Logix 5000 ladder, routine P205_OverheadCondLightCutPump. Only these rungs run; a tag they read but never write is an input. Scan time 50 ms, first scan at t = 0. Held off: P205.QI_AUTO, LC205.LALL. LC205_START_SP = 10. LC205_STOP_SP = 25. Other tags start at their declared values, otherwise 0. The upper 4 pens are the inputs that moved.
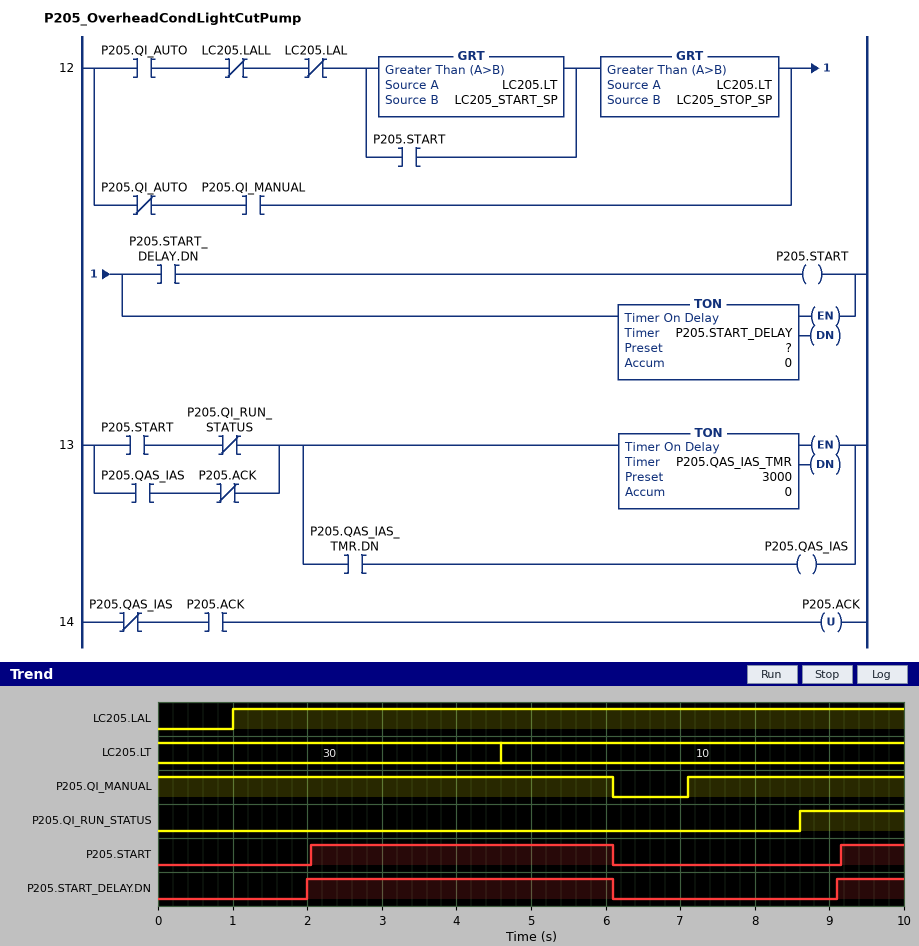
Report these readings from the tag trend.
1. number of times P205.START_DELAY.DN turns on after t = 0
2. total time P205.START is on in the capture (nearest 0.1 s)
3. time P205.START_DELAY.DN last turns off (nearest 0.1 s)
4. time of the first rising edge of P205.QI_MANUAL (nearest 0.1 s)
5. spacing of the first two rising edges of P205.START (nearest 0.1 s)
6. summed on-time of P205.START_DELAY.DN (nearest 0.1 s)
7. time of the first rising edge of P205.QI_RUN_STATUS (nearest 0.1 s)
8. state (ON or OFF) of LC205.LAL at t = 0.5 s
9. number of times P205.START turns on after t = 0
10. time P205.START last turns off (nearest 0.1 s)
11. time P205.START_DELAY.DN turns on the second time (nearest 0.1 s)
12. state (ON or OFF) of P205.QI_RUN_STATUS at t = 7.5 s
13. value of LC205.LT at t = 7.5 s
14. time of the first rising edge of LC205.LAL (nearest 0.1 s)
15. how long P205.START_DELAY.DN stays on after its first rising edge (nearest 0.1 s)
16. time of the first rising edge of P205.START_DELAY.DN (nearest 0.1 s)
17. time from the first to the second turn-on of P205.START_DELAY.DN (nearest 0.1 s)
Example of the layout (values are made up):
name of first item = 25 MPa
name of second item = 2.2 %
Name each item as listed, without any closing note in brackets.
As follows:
number of times P205.START_DELAY.DN turns on after t = 0 = 2
total time P205.START is on in the capture = 4.9 s
time P205.START_DELAY.DN last turns off = 6.1 s
time of the first rising edge of P205.QI_MANUAL = 7.1 s
spacing of the first two rising edges of P205.START = 7.1 s
summed on-time of P205.START_DELAY.DN = 5.0 s
time of the first rising edge of P205.QI_RUN_STATUS = 8.6 s
state (ON or OFF) of LC205.LAL at t = 0.5 s = OFF
number of times P205.START turns on after t = 0 = 2
time P205.START last turns off = 6.1 s
time P205.START_DELAY.DN turns on the second time = 9.1 s
state (ON or OFF) of P205.QI_RUN_STATUS at t = 7.5 s = OFF
value of LC205.LT at t = 7.5 s = 10
time of the first rising edge of LC205.LAL = 1.0 s
how long P205.START_DELAY.DN stays on after its first rising edge = 4.1 s
time of the first rising edge of P205.START_DELAY.DN = 2.0 s
time from the first to the second turn-on of P205.START_DELAY.DN = 7.1 s
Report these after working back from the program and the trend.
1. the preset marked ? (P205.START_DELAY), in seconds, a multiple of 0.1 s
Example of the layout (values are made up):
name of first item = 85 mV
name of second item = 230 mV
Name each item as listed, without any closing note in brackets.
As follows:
the preset marked ? (P205.START_DELAY), in seconds, a multiple of 0.1 s = 2.0 s
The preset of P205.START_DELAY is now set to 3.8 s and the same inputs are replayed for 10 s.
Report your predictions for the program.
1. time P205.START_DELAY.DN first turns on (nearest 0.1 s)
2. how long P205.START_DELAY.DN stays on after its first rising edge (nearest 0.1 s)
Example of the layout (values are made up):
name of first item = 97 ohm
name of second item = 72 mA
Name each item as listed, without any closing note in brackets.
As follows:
time P205.START_DELAY.DN first turns on = 3.8 s
how long P205.START_DELAY.DN stays on after its first rising edge = 2.3 s
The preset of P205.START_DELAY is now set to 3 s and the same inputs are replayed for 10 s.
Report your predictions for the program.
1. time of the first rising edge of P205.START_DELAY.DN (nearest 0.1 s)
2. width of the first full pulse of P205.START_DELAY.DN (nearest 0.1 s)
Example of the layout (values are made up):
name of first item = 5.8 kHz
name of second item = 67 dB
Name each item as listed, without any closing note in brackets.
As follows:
time of the first rising edge of P205.START_DELAY.DN = 3.0 s
width of the first full pulse of P205.START_DELAY.DN = 3.1 s
